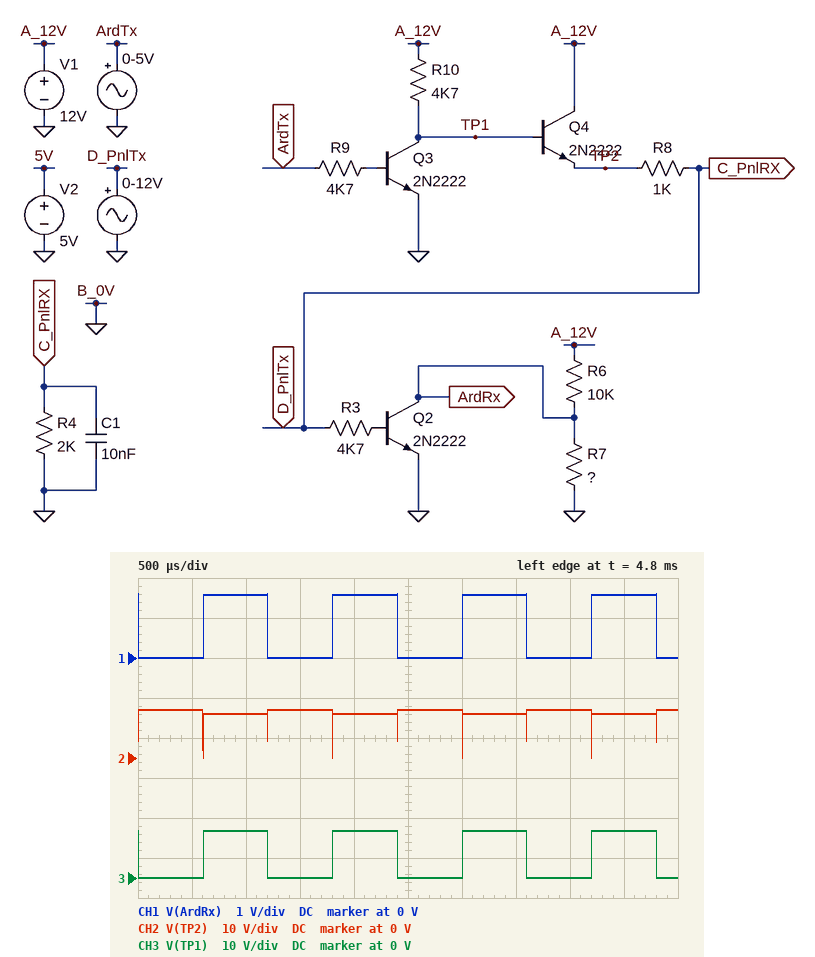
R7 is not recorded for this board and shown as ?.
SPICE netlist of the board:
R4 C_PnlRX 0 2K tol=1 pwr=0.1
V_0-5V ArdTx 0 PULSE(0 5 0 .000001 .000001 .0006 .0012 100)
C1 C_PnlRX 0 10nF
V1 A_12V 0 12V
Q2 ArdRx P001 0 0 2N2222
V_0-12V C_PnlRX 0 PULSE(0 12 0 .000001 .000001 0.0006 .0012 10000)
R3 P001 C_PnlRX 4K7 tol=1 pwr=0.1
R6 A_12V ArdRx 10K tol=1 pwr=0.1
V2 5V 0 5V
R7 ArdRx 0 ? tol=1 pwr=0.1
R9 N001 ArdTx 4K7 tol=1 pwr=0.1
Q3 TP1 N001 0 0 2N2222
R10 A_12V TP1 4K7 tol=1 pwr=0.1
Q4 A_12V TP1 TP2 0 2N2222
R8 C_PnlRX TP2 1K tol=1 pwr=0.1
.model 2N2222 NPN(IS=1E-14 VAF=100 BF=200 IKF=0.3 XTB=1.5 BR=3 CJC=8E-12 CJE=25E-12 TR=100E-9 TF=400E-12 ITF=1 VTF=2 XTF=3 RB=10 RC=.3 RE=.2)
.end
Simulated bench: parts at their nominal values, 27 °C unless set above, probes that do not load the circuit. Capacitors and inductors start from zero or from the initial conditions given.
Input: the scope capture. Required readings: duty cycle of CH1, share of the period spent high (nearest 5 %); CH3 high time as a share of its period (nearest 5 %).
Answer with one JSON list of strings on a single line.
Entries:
["50 %", "50 %"]
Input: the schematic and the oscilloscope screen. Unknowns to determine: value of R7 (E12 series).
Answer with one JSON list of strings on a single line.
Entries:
["1.5 kΩ"]
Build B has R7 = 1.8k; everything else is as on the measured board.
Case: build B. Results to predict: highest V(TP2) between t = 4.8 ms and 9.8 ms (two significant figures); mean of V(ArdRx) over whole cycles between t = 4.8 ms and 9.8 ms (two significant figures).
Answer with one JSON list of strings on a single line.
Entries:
["12 V", "920 mV"]
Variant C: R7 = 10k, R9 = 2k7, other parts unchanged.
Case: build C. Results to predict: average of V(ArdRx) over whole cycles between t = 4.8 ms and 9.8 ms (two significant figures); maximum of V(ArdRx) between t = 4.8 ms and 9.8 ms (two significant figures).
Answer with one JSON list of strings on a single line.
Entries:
["3.0 V", "6.1 V"]
